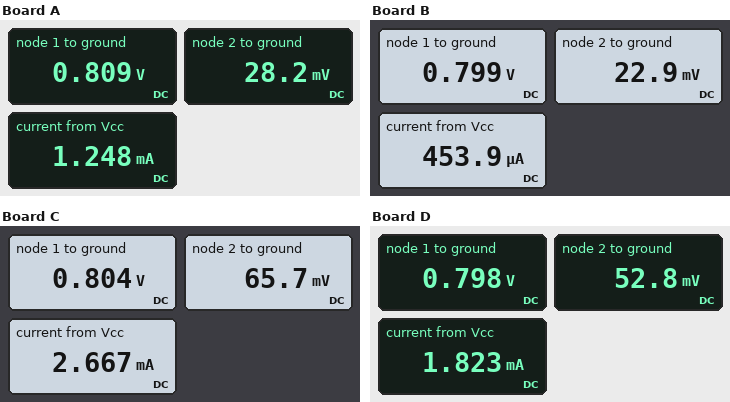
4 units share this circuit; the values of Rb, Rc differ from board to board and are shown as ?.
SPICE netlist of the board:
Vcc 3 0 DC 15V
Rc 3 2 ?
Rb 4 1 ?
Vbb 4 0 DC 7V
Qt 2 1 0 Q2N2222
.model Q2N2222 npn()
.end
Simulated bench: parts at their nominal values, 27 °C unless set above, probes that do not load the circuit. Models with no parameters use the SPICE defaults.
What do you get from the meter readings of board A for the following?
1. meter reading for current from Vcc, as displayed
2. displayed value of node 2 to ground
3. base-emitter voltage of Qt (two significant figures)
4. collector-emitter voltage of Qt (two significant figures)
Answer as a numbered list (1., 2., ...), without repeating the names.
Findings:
1. 1.248 mA
2. 28.2 mV
3. 810 mV
4. 28 mV
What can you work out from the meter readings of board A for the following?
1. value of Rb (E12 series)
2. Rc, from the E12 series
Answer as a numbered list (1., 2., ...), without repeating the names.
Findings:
1. 4.7 kΩ
2. 12 kΩ
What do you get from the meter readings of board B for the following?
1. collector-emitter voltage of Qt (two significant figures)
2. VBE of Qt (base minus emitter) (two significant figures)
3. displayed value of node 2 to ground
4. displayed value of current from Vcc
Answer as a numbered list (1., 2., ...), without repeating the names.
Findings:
1. 23 mV
2. 800 mV
3. 22.9 mV
4. 453.9 µA
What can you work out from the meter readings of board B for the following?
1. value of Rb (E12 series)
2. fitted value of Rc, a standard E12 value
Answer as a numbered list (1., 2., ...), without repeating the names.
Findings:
1. 5.6 kΩ
2. 33 kΩ
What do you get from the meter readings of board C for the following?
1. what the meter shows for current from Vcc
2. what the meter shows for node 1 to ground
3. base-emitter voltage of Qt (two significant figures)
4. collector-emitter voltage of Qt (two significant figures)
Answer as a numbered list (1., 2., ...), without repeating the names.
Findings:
1. 2.667 mA
2. 0.804 V
3. 800 mV
4. 66 mV
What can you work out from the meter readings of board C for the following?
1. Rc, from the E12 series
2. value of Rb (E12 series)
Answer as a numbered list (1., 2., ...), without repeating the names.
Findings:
1. 5.6 kΩ
2. 22 kΩ
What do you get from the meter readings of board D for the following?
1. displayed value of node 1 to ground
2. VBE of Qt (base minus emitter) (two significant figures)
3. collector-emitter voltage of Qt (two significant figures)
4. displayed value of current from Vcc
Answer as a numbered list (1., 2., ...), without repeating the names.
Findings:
1. 0.798 V
2. 800 mV
3. 53 mV
4. 1.823 mA
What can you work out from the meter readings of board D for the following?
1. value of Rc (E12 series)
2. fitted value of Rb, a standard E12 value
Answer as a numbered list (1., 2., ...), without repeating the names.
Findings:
1. 8.2 kΩ
2. 18 kΩ
